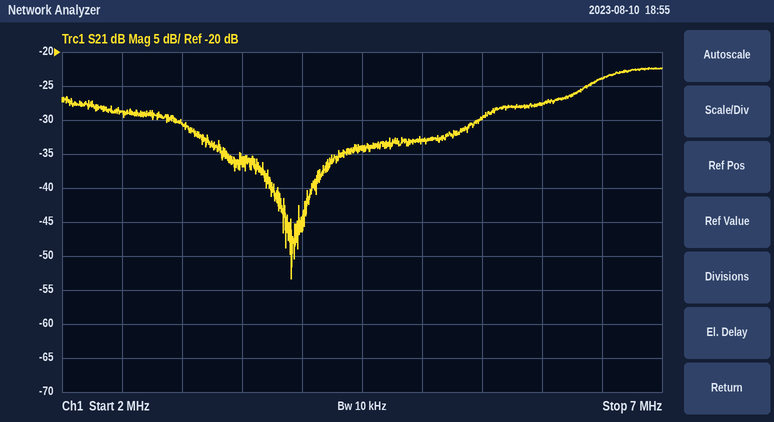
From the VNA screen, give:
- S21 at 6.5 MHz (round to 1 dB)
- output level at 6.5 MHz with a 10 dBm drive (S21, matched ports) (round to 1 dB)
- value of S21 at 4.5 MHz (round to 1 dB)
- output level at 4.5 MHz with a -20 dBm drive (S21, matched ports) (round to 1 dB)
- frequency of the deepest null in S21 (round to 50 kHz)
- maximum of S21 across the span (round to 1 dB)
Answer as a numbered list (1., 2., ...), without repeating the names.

1. -24 dB
2. -14 dBm
3. -34 dB
4. -54 dBm
5. 3.90 MHz
6. -22 dB
